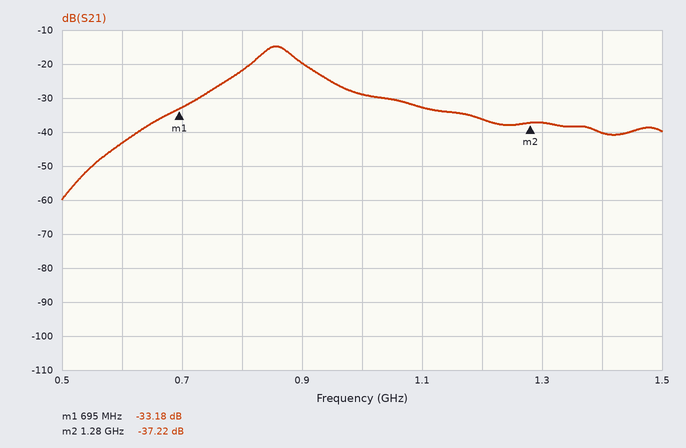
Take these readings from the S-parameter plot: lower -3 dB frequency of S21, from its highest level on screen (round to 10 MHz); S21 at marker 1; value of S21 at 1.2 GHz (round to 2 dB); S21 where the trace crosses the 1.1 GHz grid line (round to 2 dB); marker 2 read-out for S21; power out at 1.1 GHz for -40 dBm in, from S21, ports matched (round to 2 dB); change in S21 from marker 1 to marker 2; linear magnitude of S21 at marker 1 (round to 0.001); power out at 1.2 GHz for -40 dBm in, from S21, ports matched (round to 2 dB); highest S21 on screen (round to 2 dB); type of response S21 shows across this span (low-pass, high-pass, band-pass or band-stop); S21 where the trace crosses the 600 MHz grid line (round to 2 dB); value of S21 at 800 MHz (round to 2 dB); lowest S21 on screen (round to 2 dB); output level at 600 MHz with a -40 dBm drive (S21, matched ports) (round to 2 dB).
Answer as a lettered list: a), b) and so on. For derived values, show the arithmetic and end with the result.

a) 830 MHz
b) -33.18 dB
c) -36 dB
d) -32 dB
e) -37.22 dB
f) -40 dBm + (-32 dB) = -72 dBm
g) -37.22 − (-33.18) = -4.04 dB
h) 10^(-33.18/20) ≈ 0.022
i) -40 dBm + (-36 dB) = -76 dBm
j) -14 dB
k) band-pass
l) -44 dB
m) -22 dB
n) -60 dB
o) -40 dBm + (-44 dB) = -84 dBm
